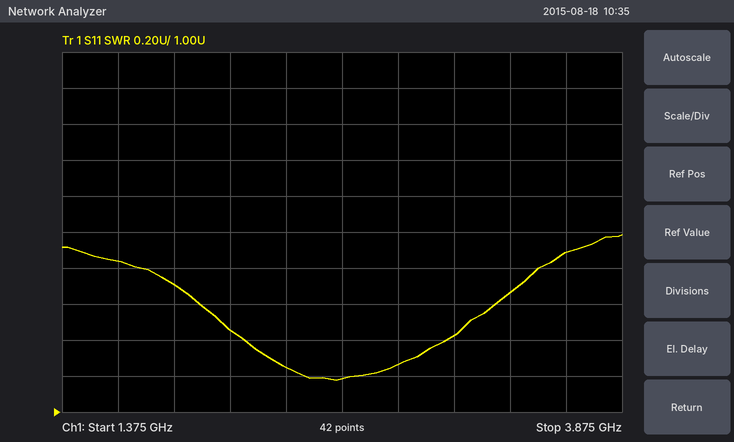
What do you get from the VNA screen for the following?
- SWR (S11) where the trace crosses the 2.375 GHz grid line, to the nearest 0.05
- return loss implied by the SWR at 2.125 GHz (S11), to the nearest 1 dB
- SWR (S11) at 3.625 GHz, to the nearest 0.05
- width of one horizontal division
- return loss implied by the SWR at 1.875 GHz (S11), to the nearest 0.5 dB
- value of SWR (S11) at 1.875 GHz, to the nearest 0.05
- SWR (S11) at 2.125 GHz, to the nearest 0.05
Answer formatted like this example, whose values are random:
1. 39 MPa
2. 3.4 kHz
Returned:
1. 1.25
2. 15 dB
3. 1.90
4. 250 MHz
5. 11.5 dB
6. 1.70
7. 1.45
